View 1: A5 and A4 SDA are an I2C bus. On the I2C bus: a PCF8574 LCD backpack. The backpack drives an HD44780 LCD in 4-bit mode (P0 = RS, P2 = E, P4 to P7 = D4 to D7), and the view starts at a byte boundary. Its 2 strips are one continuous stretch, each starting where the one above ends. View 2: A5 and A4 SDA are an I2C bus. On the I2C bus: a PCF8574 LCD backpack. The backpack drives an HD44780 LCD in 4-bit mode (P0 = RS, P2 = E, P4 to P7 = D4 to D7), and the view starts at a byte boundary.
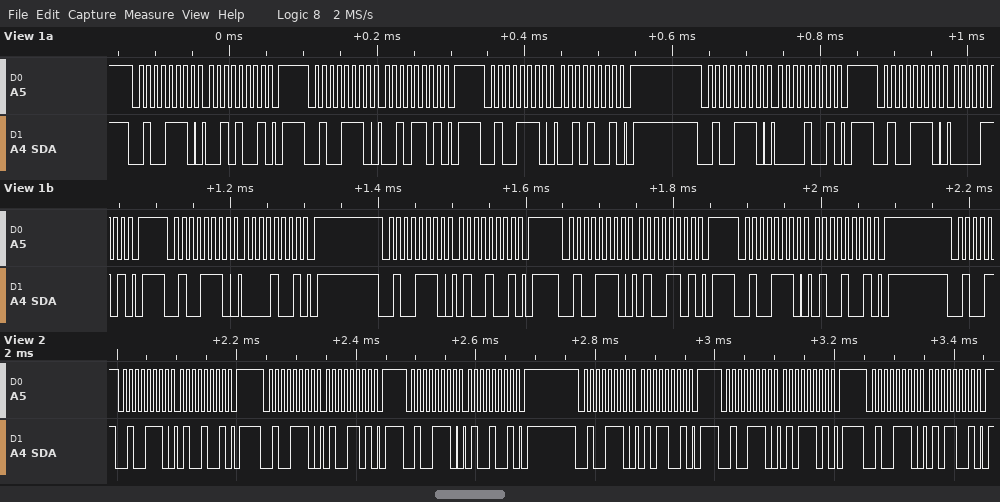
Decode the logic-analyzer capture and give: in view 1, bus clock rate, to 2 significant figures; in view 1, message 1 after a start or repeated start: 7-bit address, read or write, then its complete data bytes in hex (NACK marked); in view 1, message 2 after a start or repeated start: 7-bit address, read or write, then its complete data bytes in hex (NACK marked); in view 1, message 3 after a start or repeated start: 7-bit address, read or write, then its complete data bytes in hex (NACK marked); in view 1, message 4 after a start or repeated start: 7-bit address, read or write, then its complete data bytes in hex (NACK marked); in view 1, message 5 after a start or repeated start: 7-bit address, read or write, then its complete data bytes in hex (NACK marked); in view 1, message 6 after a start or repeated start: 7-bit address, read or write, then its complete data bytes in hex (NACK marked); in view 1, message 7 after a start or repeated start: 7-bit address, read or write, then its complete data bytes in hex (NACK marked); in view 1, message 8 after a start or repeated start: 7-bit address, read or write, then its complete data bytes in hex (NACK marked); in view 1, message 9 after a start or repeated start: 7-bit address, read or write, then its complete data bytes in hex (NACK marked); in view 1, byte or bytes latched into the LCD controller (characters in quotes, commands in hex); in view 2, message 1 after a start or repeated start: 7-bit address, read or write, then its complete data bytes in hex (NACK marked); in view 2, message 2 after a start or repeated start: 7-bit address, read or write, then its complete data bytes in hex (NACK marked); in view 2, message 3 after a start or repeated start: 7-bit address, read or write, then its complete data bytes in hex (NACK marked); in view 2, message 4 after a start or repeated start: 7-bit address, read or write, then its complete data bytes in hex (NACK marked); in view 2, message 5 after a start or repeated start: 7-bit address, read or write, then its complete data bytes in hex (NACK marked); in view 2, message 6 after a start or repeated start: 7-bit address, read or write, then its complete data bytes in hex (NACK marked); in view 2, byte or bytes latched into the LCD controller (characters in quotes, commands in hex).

100 kHz
0x27 write: 29
0x27 write: 2D
0x27 write: 29
0x27 write: 09
0x27 write: 0D
0x27 write: 09
0x27 write: 49
0x27 write: 4D
0x27 write: 49
' '
0x27 write: 49
0x27 write: 4D
0x27 write: 49
0x27 write: 59
0x27 write: 5D
0x27 write: 59
'E'
